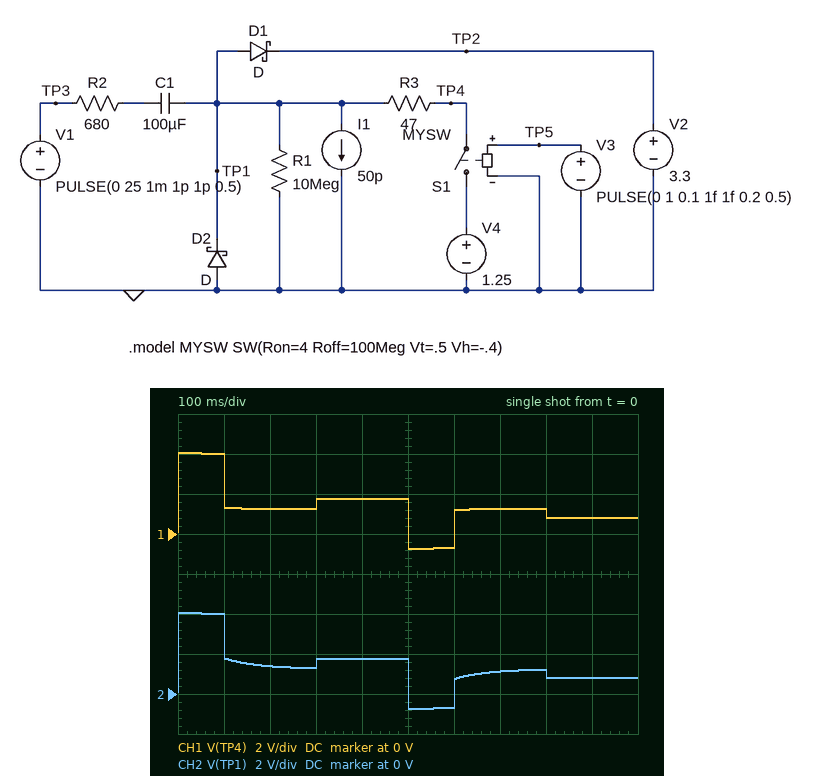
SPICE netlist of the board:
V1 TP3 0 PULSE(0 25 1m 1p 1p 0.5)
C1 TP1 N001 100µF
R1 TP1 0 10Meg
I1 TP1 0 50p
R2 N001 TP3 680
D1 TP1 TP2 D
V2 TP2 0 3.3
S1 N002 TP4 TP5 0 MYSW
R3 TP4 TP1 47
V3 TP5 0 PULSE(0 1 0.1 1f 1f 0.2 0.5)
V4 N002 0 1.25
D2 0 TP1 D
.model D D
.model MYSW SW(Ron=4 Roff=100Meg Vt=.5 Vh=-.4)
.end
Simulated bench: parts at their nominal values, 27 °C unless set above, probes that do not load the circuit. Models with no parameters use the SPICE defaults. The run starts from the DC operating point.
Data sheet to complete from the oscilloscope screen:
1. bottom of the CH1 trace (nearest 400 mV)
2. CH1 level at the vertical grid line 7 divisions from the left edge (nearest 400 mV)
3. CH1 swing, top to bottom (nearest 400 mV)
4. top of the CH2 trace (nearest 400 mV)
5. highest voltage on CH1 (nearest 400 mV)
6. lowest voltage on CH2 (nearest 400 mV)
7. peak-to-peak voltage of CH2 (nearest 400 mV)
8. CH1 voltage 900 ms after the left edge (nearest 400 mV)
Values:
-800 mV
1.2 V
4.8 V
4.0 V
4.0 V
-800 mV
4.8 V
800 mV
